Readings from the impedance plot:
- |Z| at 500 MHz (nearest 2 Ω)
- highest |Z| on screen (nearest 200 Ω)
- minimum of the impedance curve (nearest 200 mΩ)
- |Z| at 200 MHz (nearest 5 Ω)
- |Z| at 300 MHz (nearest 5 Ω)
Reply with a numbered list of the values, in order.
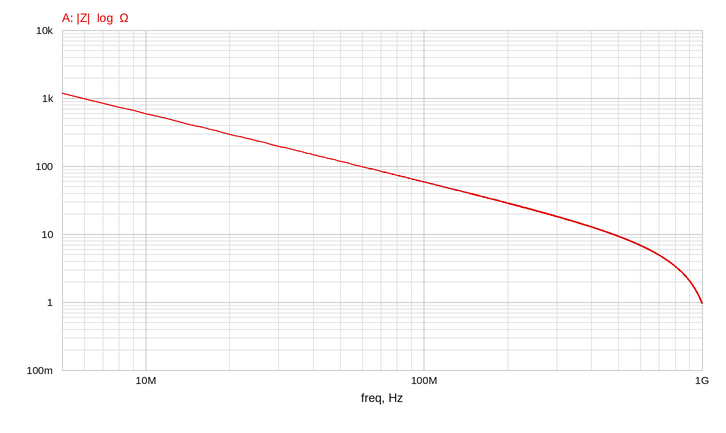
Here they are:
1. 10 Ω
2. 1.2 kΩ
3. 1.0 Ω
4. 30 Ω
5. 20 Ω
